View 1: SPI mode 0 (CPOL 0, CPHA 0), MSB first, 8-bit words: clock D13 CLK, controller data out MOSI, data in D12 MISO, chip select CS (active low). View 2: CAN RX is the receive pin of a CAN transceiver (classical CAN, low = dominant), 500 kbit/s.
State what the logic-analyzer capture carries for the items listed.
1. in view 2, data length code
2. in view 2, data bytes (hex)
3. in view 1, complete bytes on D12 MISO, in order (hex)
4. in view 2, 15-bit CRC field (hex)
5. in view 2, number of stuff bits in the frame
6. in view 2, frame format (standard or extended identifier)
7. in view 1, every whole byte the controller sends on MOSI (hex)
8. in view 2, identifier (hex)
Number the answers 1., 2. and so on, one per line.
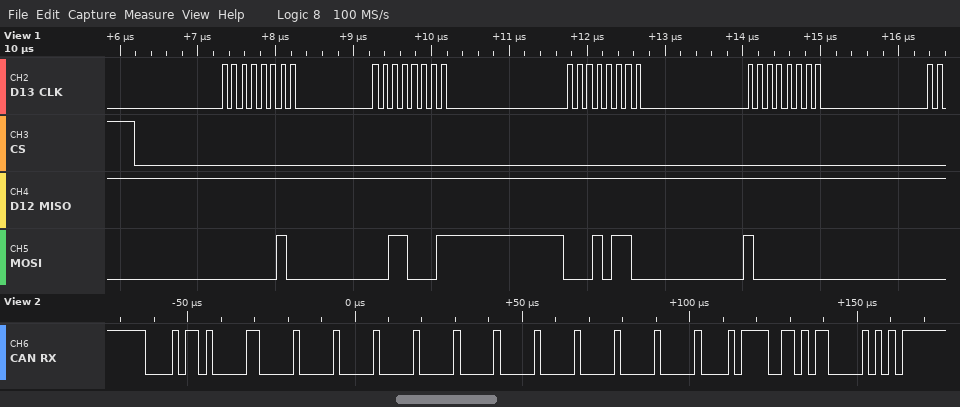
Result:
1. 8
2. 00 00 00 00 00 00 00 BC
3. FF FF FF FF
4. 0x6B02
5. 13
6. standard
7. 02 31 16 80
8. 0x0B4
